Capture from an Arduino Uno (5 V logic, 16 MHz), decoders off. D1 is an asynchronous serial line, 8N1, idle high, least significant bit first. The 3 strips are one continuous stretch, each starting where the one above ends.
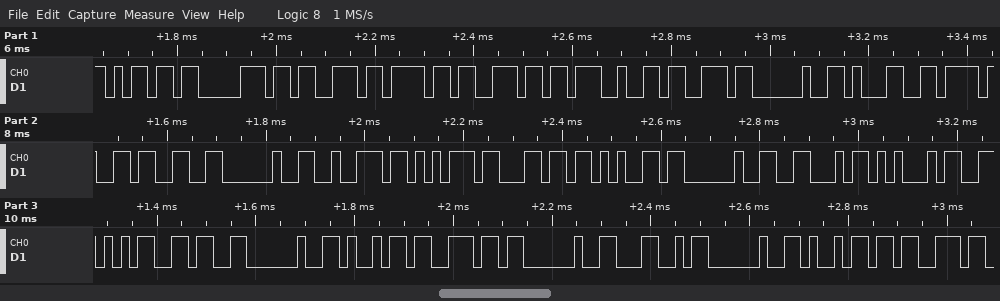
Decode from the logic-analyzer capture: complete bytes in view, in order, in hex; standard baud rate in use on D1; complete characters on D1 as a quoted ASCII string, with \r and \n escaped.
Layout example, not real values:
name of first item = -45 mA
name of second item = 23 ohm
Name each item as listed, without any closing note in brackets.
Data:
complete bytes in view, in order, in hex = 6D 70 73 6F 6E 27 73 20 31 2F 33 20 72 75 6C 65 20 46 45 56 36 20 69 6E 20 4C 20 69 73
standard baud rate in use on D1 = 57600 baud
complete characters on D1 as a quoted ASCII string, with \r and \n escaped = "mpson's 1/3 rule FEV6 in L is"
